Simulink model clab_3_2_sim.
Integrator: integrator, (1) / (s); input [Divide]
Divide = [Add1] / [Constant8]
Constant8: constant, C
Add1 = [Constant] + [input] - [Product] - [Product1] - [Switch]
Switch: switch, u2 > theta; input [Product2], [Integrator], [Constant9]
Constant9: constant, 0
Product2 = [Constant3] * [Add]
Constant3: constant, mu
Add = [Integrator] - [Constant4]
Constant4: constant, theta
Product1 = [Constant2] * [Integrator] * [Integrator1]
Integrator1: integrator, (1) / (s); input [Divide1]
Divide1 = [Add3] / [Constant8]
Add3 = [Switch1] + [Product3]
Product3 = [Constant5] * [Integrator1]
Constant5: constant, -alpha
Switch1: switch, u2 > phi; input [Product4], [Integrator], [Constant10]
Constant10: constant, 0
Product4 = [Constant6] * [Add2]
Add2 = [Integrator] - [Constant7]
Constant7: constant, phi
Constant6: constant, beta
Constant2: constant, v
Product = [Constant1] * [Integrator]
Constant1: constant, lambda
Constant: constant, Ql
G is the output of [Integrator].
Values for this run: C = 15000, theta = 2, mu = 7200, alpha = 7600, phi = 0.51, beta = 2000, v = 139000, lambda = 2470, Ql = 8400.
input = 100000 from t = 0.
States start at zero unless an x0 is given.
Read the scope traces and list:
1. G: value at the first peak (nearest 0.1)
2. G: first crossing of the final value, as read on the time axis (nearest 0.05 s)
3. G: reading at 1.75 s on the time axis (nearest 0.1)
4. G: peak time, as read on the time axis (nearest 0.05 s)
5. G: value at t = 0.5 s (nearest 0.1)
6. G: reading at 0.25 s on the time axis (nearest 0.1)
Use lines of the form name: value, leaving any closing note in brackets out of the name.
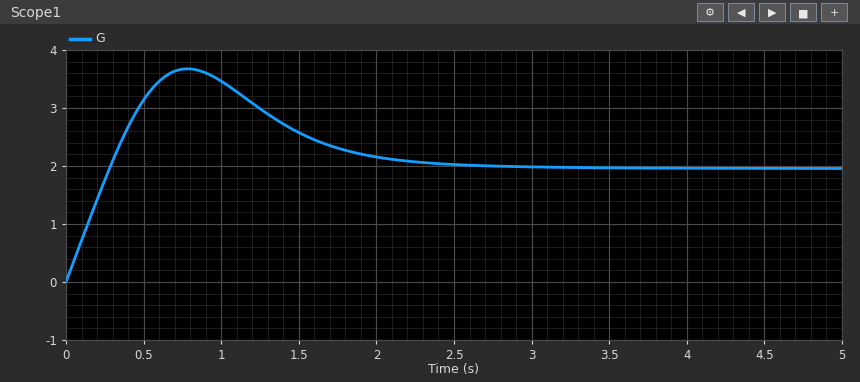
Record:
G: value at the first peak: 3.7
G: first crossing of the final value, as read on the time axis: 0.30 s
G: reading at 1.75 s on the time axis: 2.3
G: peak time, as read on the time axis: 0.80 s
G: value at t = 0.5 s: 3.1
G: reading at 0.25 s on the time axis: 1.8
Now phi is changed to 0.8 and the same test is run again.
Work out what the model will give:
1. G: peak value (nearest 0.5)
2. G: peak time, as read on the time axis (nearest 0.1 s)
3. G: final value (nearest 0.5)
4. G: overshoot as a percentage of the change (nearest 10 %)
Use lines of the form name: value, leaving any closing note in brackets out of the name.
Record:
G: peak value: 4.0
G: peak time, as read on the time axis: 0.8 s
G: final value: 2.0
G: overshoot as a percentage of the change: 80 %
